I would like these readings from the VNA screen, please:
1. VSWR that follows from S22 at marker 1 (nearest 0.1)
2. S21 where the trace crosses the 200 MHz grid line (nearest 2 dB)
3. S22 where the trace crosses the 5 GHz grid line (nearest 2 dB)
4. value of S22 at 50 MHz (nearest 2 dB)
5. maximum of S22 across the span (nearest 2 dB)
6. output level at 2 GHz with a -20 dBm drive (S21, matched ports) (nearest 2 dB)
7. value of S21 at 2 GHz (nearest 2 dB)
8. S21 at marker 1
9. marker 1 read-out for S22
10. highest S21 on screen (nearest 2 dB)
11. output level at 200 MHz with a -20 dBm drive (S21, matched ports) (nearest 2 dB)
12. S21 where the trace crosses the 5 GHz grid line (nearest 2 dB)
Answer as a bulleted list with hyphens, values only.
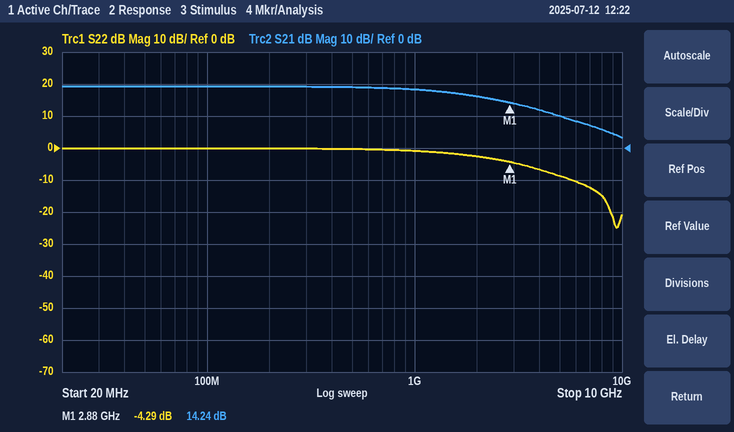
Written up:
- 4.1
- 20 dB
- -8 dB
- 0 dB
- 0 dB
- -4 dBm
- 16 dB
- 14.24 dB
- -4.29 dB
- 20 dB
- 0 dBm
- 10 dB
